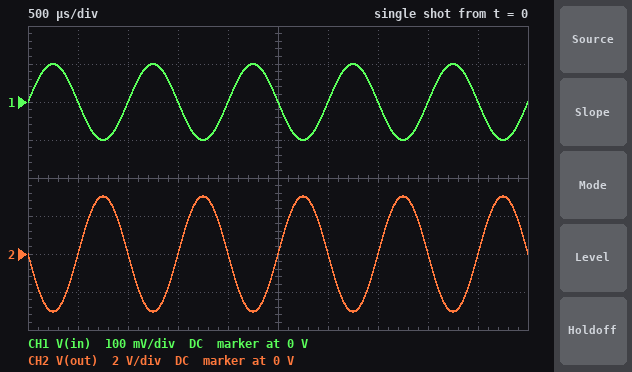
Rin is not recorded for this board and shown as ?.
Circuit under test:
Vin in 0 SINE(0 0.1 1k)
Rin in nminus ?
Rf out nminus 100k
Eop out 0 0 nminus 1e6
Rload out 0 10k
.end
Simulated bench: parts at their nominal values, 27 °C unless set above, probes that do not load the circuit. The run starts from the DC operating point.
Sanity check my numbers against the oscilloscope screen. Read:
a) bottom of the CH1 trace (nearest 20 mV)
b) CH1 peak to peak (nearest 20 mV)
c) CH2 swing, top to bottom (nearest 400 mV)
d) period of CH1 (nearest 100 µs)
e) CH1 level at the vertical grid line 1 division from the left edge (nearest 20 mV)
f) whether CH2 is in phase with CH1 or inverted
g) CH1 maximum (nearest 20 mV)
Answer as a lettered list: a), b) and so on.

a) -100 mV
b) 200 mV
c) 6.0 V
d) 1.0 ms
e) 0 V
f) inverted
g) 100 mV
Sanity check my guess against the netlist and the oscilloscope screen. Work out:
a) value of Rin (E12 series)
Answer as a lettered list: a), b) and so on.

a) 3.3 kΩ
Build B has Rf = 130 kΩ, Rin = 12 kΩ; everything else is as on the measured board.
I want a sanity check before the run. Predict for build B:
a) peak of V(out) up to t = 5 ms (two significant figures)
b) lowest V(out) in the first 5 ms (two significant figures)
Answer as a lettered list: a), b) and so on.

a) 1.1 V
b) -1.1 V
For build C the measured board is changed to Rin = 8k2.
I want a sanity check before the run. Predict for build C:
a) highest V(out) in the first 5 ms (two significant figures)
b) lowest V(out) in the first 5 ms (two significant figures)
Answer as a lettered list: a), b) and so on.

a) 1.2 V
b) -1.2 V
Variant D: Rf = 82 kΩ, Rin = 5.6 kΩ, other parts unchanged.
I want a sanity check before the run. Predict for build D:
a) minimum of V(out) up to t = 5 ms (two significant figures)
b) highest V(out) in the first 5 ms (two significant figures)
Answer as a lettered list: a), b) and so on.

a) -1.5 V
b) 1.5 V
